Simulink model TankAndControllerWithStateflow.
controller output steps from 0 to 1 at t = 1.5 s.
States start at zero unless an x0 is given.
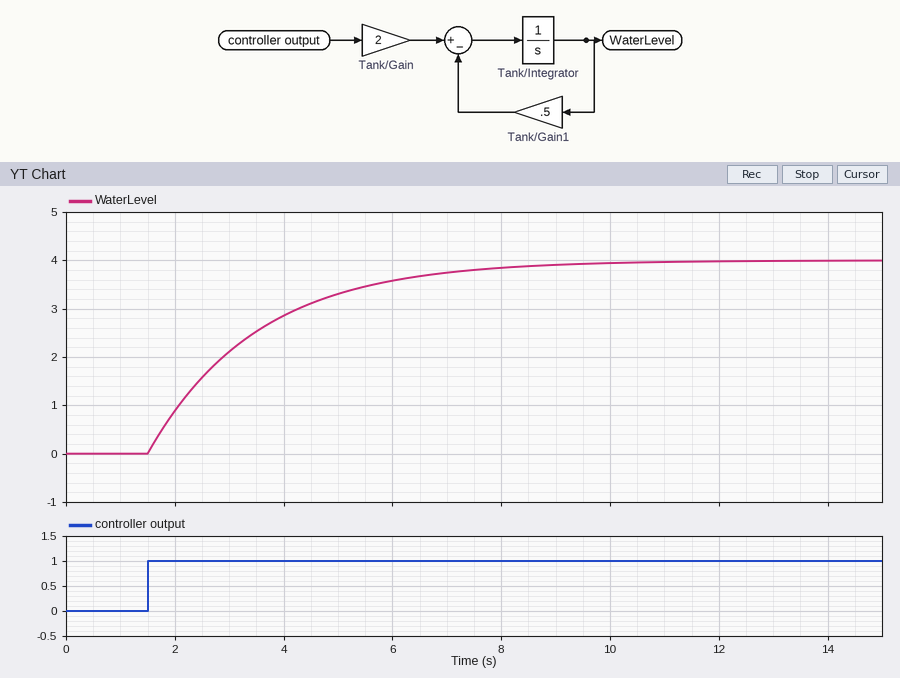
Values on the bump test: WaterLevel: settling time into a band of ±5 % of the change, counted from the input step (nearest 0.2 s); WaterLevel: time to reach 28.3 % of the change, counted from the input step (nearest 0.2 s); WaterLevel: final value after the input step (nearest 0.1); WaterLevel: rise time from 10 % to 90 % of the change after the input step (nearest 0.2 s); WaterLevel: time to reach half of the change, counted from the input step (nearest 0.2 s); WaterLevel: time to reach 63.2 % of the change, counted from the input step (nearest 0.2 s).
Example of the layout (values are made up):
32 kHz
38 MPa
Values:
6.0 s
0.6 s
4.0
4.4 s
1.4 s
2.0 s
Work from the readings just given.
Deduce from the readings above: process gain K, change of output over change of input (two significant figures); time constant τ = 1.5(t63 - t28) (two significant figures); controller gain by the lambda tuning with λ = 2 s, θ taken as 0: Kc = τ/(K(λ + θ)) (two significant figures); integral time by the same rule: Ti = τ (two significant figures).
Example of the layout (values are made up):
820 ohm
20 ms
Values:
4.0
2.1 s
0.26
2.1 s
